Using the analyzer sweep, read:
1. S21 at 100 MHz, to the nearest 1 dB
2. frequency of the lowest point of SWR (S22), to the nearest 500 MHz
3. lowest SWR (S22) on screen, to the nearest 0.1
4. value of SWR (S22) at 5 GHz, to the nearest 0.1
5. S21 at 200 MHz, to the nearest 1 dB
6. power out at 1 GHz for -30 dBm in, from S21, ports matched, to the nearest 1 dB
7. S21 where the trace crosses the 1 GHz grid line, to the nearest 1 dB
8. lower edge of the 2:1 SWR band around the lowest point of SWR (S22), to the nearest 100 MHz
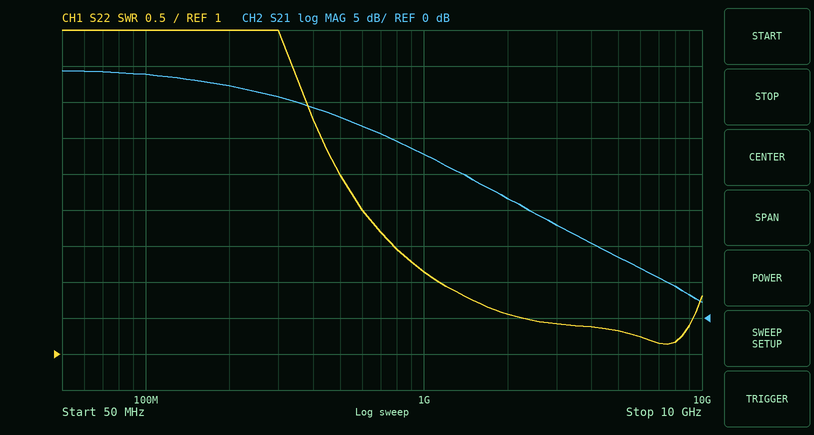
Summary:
34 dB
7.5 GHz
1.1
1.3
32 dB
-7 dBm
23 dB
1.1 GHz
